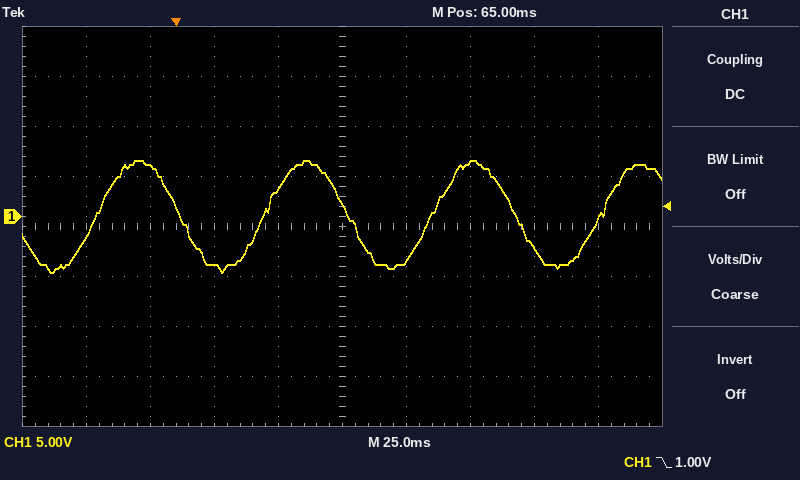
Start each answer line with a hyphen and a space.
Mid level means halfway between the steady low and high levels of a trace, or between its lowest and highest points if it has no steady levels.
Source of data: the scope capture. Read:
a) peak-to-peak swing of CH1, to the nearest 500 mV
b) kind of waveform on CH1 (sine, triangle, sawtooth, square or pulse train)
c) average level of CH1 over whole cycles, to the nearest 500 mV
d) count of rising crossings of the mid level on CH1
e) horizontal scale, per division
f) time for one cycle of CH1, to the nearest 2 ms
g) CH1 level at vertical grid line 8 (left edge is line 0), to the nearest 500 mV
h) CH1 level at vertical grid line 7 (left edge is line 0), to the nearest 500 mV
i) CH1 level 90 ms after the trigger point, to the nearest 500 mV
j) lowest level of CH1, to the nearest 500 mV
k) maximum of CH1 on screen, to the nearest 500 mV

- 11.0 V
- sine
- 0.0 V
- 4
- 25 ms
- 66 ms
- -3.0 V
- 5.5 V
- -4.5 V
- -5.5 V
- 5.5 V
